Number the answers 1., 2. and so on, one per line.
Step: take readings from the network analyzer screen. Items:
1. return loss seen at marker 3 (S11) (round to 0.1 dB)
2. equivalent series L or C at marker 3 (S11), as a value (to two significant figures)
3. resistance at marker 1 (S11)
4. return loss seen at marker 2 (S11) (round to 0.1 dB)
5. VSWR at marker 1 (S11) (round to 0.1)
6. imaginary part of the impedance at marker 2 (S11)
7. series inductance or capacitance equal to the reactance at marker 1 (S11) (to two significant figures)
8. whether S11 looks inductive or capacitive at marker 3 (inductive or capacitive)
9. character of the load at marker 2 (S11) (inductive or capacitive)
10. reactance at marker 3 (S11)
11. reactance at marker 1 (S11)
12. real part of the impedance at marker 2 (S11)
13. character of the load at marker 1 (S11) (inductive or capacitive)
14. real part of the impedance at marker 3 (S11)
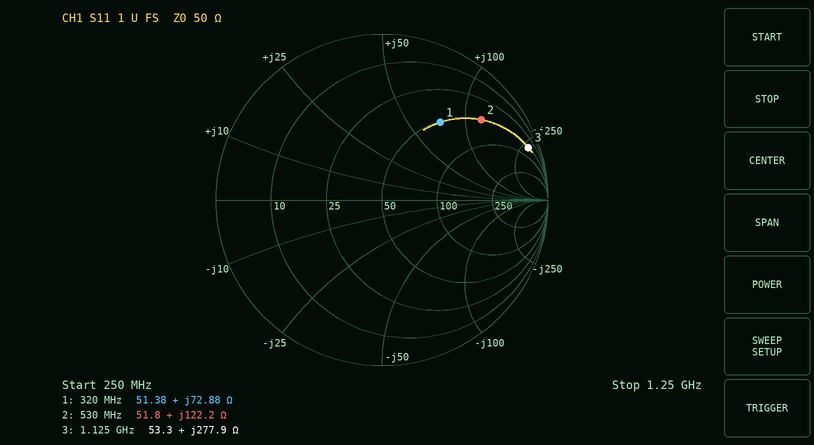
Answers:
1. 0.6 dB
2. 39 nH
3. 51.38 Ω
4. 2.3 dB
5. 3.8
6. +122.2 Ω
7. 36 nH
8. inductive
9. inductive
10. +277.9 Ω
11. +72.88 Ω
12. 51.8 Ω
13. inductive
14. 53.3 Ω
